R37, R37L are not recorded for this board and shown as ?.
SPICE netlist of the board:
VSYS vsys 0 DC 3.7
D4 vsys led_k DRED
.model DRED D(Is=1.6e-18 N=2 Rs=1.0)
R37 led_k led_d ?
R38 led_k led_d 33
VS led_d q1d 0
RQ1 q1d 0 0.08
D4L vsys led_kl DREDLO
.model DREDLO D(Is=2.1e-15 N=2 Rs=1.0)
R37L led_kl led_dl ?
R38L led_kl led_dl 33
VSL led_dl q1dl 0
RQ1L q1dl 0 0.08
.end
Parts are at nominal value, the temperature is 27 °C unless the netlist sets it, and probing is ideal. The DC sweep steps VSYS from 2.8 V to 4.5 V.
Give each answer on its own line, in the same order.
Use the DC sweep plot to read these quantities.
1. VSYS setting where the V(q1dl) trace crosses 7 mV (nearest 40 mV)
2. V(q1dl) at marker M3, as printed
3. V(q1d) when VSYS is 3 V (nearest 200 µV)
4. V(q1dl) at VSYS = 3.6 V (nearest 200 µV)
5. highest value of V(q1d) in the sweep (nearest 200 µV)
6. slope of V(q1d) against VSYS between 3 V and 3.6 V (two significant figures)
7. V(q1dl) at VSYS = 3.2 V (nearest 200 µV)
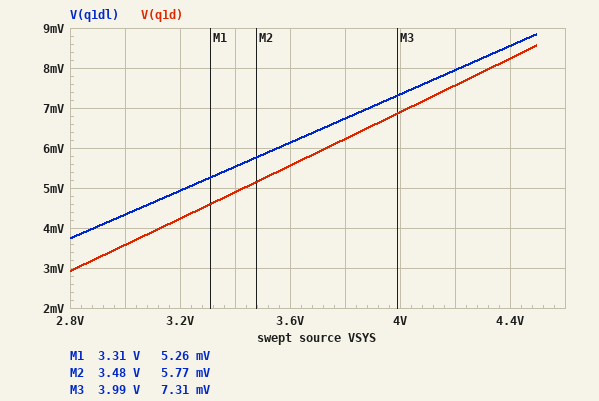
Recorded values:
3.88 V
7.31 mV
3.6 mV
6.2 mV
8.6 mV
0.0033 V/V
5.0 mV
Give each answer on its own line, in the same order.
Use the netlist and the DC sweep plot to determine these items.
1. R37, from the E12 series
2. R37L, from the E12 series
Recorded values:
68 Ω
100 Ω
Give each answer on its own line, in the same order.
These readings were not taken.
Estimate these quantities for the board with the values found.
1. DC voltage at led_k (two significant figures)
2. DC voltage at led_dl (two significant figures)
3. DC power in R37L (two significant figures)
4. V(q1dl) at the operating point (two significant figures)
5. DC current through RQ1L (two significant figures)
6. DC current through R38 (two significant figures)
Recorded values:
1.6 V
6.4 mV
40 mW
6.4 mV
80 mA
50 mA
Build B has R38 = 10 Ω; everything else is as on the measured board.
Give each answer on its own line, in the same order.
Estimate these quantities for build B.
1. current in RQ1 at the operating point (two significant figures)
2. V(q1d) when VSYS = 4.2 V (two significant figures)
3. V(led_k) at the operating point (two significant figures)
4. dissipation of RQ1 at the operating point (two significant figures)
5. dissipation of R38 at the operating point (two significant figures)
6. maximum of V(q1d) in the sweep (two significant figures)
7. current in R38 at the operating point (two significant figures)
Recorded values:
170 mA
18 mV
1.5 V
2.3 mW
220 mW
20 mV
150 mA
